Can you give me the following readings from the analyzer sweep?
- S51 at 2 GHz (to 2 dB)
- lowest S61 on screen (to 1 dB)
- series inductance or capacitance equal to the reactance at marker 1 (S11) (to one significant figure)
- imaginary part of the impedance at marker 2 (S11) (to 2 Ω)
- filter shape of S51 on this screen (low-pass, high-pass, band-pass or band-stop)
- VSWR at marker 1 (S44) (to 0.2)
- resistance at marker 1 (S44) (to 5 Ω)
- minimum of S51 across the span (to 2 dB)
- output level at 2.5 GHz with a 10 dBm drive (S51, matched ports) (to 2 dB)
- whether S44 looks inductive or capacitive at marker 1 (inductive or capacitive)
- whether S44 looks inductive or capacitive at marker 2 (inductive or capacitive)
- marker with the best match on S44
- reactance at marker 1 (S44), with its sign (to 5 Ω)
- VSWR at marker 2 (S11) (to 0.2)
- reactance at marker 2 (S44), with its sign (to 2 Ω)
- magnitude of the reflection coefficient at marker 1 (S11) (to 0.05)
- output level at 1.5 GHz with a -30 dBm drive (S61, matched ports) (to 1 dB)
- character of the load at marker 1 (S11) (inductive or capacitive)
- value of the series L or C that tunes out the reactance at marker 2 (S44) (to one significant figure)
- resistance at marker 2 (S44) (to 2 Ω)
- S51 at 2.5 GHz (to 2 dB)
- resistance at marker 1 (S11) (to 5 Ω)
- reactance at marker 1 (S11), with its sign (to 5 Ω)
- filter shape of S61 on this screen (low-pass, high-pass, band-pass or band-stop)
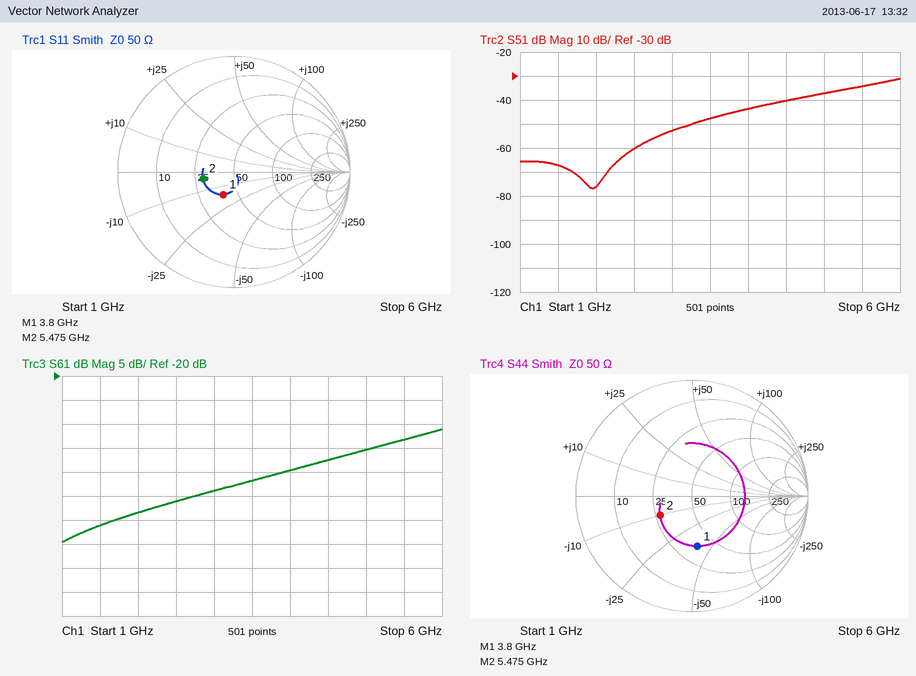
-76 dB
-55 dB
3 pF
-4 Ω
high-pass
2.6
35 Ω
-76 dB
-50 dBm
capacitive
capacitive
marker 2
-40 Ω
1.8
-10 Ω
0.20
-81 dBm
capacitive
300 pH
28 Ω
-60 dB
40 Ω
-15 Ω
high-pass
